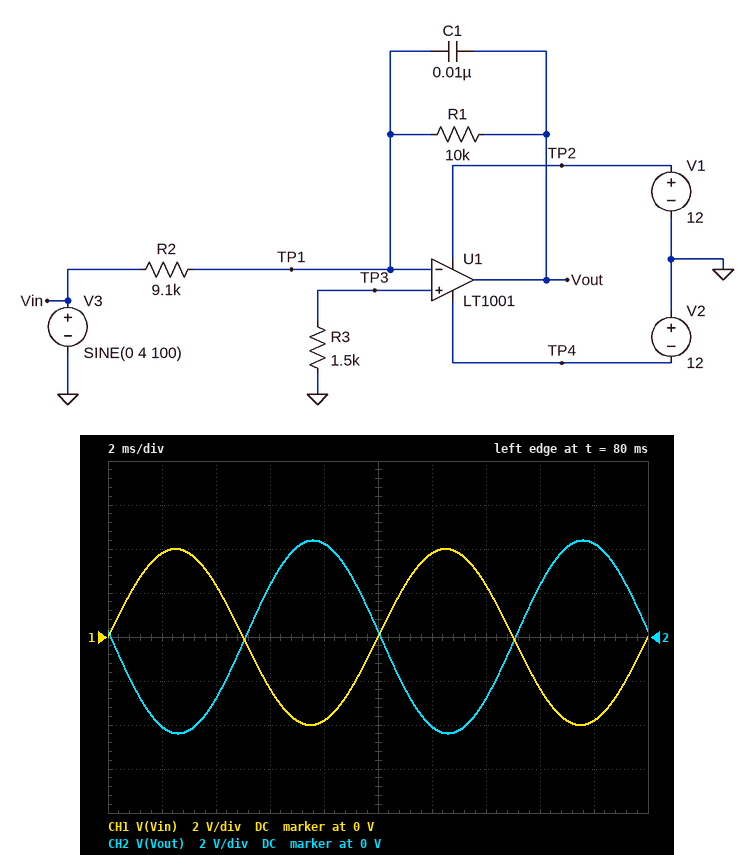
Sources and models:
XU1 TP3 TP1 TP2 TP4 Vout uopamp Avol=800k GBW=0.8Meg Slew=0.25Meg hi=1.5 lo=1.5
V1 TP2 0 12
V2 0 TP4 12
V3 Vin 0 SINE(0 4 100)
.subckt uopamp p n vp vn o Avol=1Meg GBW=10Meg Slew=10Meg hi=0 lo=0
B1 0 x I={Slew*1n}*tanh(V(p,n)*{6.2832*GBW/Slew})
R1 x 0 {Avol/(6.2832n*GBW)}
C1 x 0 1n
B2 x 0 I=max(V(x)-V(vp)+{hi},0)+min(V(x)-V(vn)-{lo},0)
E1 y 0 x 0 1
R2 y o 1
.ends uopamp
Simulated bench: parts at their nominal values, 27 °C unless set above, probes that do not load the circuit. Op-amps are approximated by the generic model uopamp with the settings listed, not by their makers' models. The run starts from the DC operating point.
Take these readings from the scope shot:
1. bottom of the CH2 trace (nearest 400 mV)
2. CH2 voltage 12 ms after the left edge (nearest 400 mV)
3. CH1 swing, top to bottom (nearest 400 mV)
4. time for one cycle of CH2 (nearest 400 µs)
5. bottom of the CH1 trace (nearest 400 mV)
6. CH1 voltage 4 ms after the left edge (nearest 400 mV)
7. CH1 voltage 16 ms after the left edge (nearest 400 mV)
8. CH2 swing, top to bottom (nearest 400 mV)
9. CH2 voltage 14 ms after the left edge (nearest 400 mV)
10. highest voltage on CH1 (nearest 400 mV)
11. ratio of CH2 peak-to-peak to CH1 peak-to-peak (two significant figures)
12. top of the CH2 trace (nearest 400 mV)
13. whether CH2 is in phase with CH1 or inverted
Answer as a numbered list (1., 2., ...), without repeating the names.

1. -4.4 V
2. -4.0 V
3. 8.0 V
4. 10.0 ms
5. -4.0 V
6. 2.4 V
7. -2.4 V
8. 8.8 V
9. -2.8 V
10. 4.0 V
11. 1.1
12. 4.4 V
13. inverted
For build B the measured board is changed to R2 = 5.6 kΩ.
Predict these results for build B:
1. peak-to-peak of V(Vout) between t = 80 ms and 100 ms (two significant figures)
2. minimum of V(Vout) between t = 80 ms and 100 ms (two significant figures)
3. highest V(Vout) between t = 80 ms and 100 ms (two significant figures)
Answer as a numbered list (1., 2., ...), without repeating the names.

1. 14 V
2. -7.1 V
3. 7.1 V
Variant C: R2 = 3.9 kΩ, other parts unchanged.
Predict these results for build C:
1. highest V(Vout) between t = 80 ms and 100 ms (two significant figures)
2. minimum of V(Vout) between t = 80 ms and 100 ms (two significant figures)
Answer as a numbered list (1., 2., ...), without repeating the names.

1. 10 V
2. -10 V
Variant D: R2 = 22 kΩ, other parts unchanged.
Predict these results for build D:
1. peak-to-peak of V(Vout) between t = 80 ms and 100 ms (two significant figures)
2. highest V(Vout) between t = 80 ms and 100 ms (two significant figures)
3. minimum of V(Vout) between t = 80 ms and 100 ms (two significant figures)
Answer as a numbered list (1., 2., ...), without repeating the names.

1. 3.6 V
2. 1.8 V
3. -1.8 V
